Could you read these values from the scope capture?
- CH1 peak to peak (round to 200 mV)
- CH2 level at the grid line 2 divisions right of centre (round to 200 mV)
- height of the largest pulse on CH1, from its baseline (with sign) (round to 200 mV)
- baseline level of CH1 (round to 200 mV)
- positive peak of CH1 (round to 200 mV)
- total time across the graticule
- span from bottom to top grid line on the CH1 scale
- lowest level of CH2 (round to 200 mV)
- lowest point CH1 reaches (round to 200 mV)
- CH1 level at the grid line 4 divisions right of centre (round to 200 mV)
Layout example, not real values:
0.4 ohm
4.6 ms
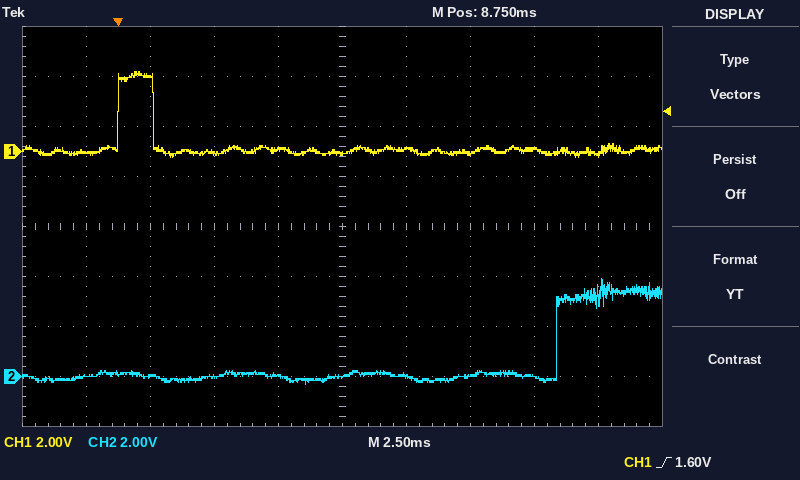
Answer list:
3.4 V
0.0 V
+3.2 V
0.0 V
3.2 V
25 ms
16 V
-400 mV
-200 mV
-200 mV
